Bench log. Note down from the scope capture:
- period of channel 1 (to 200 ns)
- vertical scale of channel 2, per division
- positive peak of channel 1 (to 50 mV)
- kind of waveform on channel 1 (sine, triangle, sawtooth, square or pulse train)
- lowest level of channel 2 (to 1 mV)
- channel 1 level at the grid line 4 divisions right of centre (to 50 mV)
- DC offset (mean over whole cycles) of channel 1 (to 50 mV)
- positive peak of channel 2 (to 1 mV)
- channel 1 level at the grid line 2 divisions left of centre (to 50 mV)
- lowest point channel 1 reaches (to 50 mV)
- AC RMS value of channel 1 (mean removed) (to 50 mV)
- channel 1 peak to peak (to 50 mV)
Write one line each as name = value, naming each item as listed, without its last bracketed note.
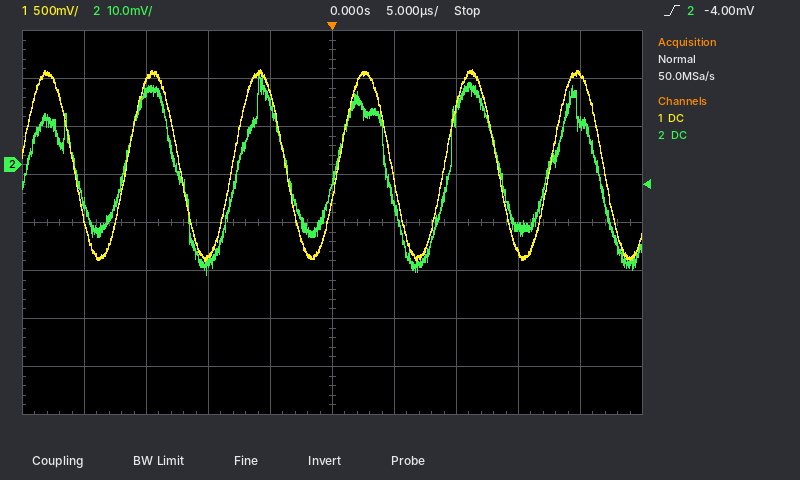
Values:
period of channel 1 = 8.6 µs
vertical scale of channel 2, per division = 10 mV
positive peak of channel 1 = 1.00 V
kind of waveform on channel 1 = sine
lowest level of channel 2 = -23 mV
channel 1 level at the grid line 4 divisions right of centre = 950 mV
DC offset (mean over whole cycles) of channel 1 = 0 mV
positive peak of channel 2 = 19 mV
channel 1 level at the grid line 2 divisions left of centre = -950 mV
lowest point channel 1 reaches = -1.00 V
AC RMS value of channel 1 (mean removed) = 700 mV
channel 1 peak to peak = 2.00 V
